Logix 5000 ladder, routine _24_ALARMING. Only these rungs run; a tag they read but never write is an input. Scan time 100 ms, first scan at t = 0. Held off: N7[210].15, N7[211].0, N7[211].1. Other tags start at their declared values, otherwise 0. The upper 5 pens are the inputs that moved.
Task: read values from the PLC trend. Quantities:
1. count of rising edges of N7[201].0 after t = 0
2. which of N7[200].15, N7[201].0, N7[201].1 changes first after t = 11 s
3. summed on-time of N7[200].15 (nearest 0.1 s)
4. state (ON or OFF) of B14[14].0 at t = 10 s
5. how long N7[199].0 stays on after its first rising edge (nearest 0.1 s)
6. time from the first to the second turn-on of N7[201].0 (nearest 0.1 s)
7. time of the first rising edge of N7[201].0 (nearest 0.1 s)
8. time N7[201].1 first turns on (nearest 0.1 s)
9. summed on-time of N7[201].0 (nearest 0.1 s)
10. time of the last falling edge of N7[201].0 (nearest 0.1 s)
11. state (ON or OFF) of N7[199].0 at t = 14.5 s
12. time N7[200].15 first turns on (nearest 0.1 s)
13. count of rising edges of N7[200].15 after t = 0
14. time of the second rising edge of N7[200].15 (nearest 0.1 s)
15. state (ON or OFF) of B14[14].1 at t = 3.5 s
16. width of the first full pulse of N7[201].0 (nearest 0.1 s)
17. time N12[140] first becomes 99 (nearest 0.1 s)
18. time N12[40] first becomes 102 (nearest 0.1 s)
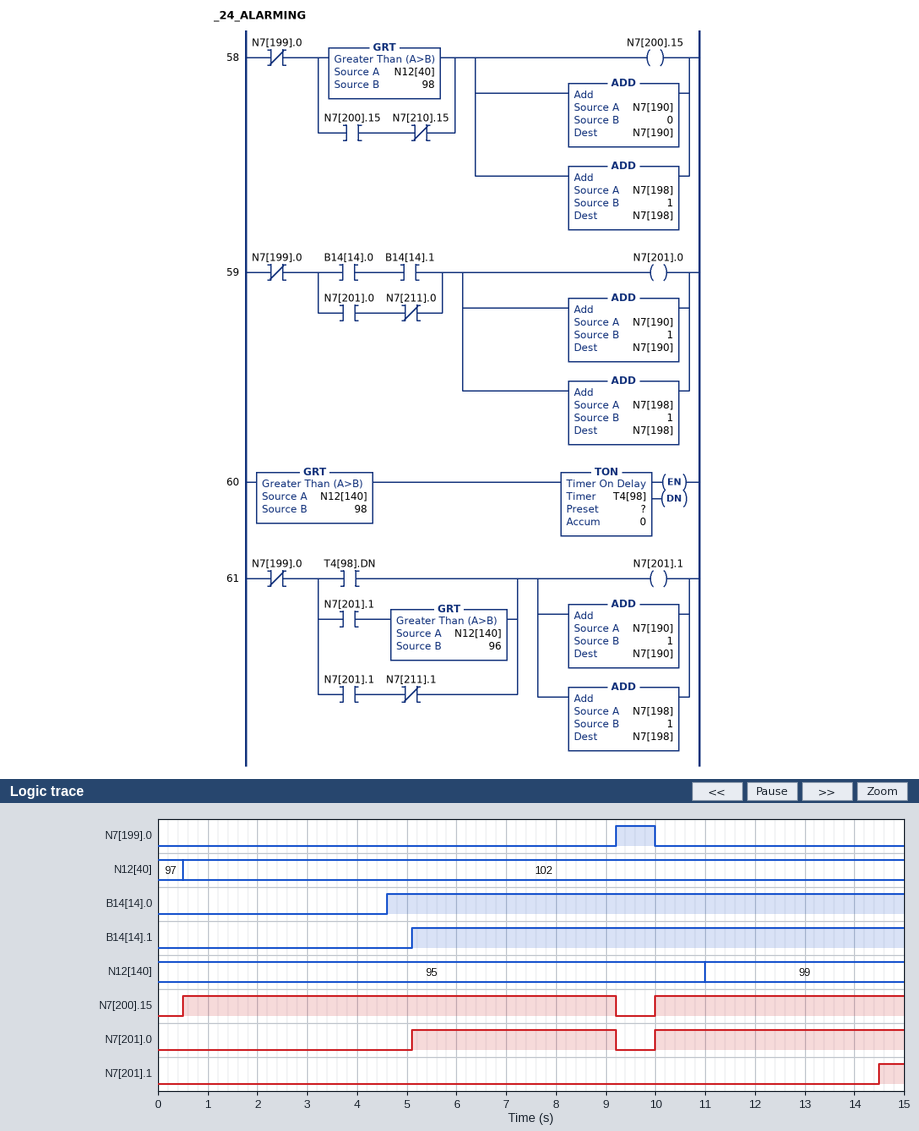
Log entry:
2
N7[201].1
13.7 s
ON
0.8 s
4.9 s
5.1 s
14.5 s
9.1 s
9.2 s
OFF
0.5 s
2
10.0 s
OFF
4.1 s
11.0 s
0.5 s
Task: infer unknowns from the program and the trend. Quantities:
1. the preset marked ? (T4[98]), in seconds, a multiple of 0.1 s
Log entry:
3.5 s
